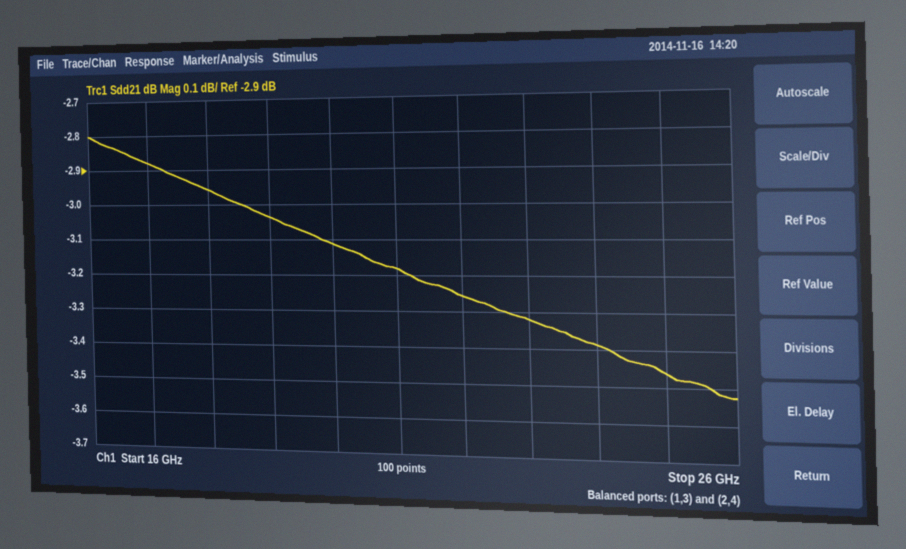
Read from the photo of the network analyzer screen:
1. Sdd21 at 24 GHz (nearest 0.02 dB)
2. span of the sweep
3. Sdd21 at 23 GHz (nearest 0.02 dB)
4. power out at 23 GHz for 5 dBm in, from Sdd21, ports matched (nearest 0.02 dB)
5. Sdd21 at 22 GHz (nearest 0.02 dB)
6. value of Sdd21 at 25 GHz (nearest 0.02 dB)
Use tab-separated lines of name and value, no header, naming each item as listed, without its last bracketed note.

Sdd21 at 24 GHz	-3.38 dB
span of the sweep	10 GHz
Sdd21 at 23 GHz	-3.32 dB
power out at 23 GHz for 5 dBm in, from Sdd21, ports matched	1.68 dBm
Sdd21 at 22 GHz	-3.26 dB
value of Sdd21 at 25 GHz	-3.46 dB
